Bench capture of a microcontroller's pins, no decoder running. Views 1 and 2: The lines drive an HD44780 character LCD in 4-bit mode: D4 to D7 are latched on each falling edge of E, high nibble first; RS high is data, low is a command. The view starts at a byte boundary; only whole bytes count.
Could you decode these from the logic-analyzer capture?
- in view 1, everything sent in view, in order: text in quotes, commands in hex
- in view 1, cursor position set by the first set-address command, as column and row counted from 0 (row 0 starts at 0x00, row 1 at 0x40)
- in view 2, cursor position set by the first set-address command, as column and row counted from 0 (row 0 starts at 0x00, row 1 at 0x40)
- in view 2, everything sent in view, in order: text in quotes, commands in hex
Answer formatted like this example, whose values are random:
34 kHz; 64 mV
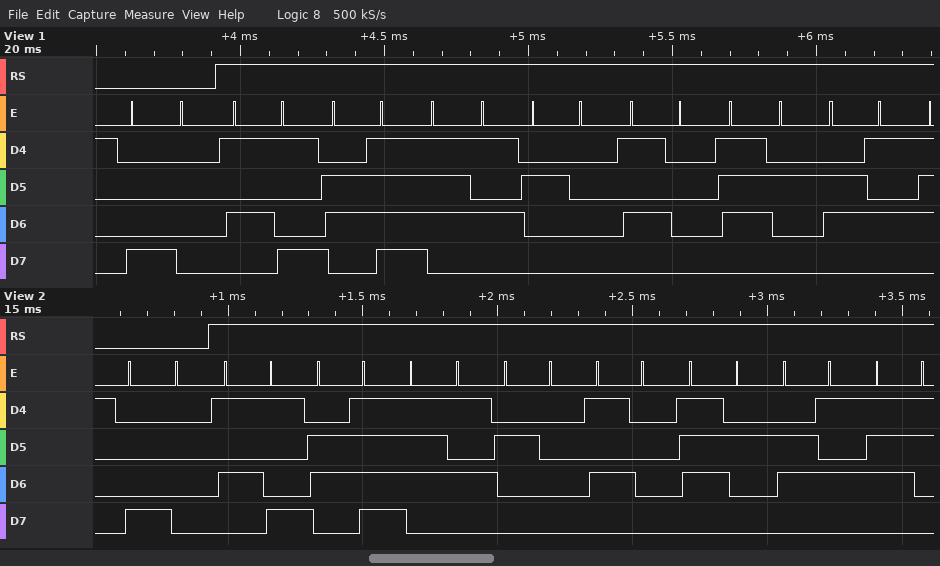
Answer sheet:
0x80 "You Pre"; column 0, row 0; column 0, row 0; 0x80 "You Pres"
